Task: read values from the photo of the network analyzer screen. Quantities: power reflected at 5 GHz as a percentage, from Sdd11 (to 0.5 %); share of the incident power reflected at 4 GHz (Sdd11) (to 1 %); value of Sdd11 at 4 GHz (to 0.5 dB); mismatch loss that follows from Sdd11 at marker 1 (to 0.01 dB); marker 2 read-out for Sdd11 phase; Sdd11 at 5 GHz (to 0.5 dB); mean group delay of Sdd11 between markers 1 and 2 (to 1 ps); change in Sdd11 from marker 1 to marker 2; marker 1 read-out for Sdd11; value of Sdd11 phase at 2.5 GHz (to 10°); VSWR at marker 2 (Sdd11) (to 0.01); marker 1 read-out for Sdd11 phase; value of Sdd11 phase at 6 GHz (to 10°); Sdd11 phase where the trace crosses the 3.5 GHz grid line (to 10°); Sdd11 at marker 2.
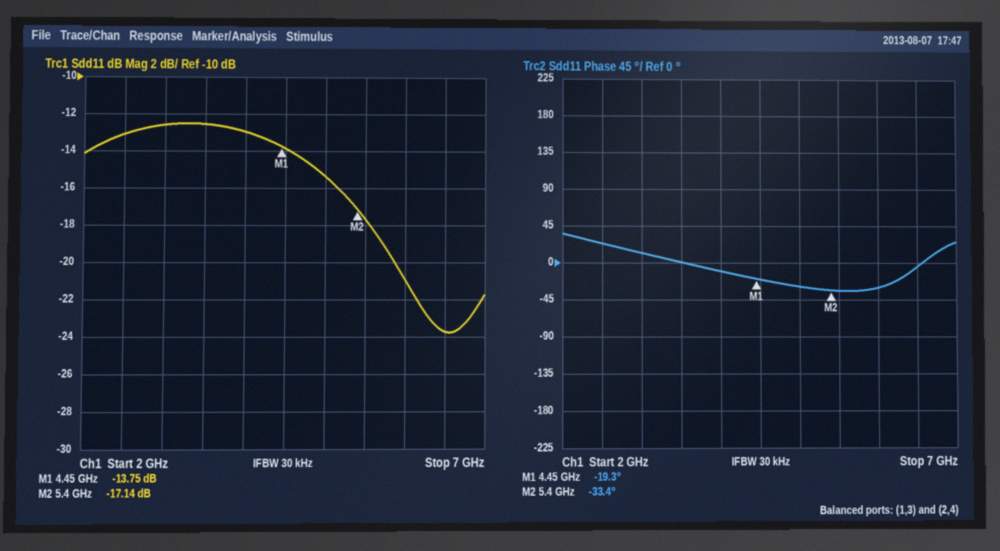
3.0 %
5 %
-13.0 dB
0.19 dB
-33.4°
-15.5 dB
41 ps
-3.39 dB
-13.75 dB
20°
1.32
-19.3°
-30°
0°
-17.14 dB
